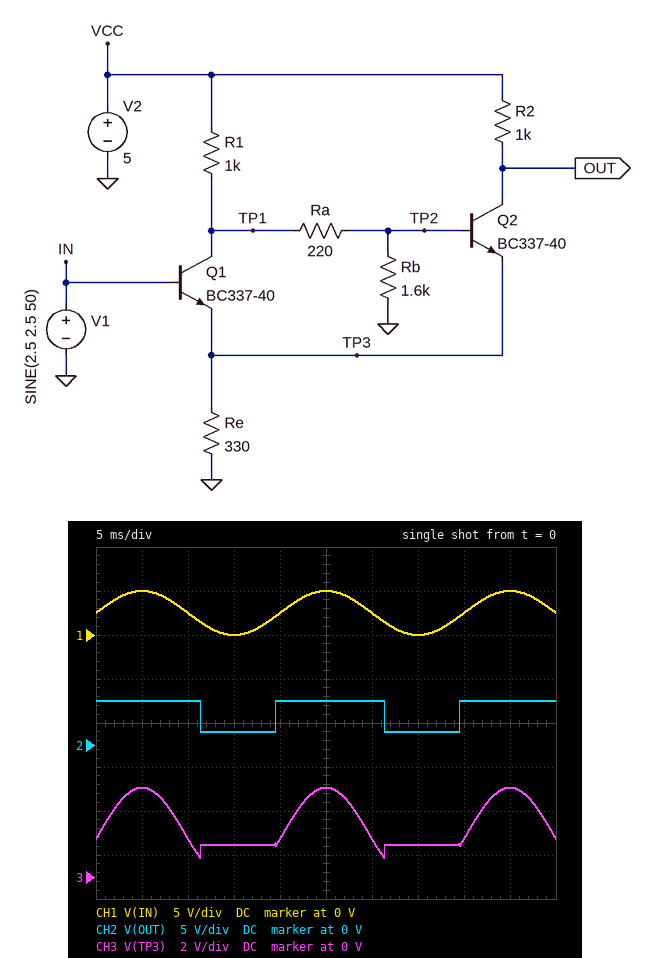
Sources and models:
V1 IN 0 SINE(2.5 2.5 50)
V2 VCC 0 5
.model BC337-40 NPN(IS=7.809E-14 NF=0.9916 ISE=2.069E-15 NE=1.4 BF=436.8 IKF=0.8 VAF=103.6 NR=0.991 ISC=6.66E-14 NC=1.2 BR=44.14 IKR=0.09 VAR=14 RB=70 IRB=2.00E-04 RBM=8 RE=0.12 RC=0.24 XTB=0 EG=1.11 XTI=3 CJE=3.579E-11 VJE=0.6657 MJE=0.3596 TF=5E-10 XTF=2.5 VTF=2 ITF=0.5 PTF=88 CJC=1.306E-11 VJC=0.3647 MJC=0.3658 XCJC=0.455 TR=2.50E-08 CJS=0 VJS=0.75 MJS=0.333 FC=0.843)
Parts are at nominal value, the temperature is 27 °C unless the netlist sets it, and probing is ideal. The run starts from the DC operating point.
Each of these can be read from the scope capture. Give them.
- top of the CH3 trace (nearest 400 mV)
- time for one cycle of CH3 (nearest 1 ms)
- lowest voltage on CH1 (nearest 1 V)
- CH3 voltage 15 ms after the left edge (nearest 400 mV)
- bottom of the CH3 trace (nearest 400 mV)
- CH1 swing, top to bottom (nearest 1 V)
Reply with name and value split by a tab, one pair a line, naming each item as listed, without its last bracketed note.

top of the CH3 trace	4.0 V
time for one cycle of CH3	20 ms
lowest voltage on CH1	0 V
CH3 voltage 15 ms after the left edge	1.6 V
bottom of the CH3 trace	800 mV
CH1 swing, top to bottom	5 V
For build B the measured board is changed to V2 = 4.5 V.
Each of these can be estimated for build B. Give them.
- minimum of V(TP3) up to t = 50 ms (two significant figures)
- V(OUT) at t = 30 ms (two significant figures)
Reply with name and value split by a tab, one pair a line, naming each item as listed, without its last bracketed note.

minimum of V(TP3) up to t = 50 ms	760 mV
V(OUT) at t = 30 ms	4.5 V
